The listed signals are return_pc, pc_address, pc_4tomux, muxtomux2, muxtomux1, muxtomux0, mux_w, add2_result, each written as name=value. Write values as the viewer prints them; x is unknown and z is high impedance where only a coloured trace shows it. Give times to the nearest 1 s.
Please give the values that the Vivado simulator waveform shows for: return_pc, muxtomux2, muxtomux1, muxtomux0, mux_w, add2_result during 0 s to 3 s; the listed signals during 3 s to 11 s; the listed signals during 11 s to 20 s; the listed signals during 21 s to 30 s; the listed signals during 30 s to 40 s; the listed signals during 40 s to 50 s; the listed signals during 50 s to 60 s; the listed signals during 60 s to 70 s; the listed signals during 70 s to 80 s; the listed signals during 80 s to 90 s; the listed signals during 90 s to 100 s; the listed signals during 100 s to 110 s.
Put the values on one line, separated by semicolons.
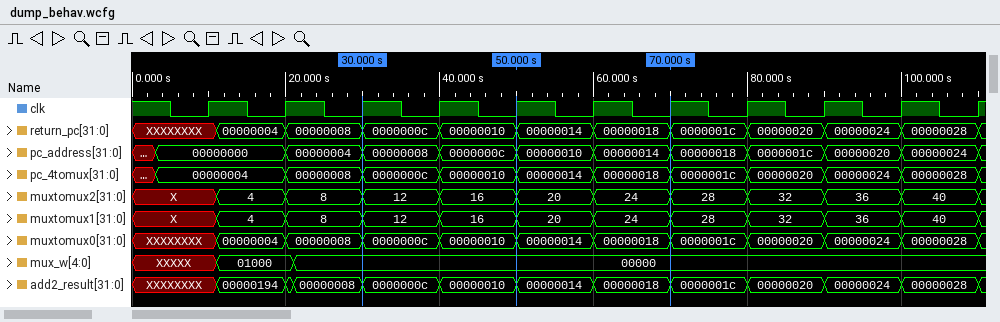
return_pc=XXXXXXXX, muxtomux2=X, muxtomux1=X, muxtomux0=XXXXXXXX, mux_w=XXXXX, add2_result=XXXXXXXX; return_pc=XXXXXXXX, pc_address=00000000, pc_4tomux=00000004, muxtomux2=X, muxtomux1=X, muxtomux0=XXXXXXXX, mux_w=XXXXX, add2_result=XXXXXXXX; return_pc=00000004, pc_address=00000000, pc_4tomux=00000004, muxtomux2=4, muxtomux1=4, muxtomux0=00000004, mux_w=01000, add2_result=00000194; return_pc=00000008, pc_address=00000004, pc_4tomux=00000008, muxtomux2=8, muxtomux1=8, muxtomux0=00000008, mux_w=00000, add2_result=00000008; return_pc=0000000c, pc_address=00000008, pc_4tomux=0000000c, muxtomux2=12, muxtomux1=12, muxtomux0=0000000c, mux_w=00000, add2_result=0000000c; return_pc=00000010, pc_address=0000000c, pc_4tomux=00000010, muxtomux2=16, muxtomux1=16, muxtomux0=00000010, mux_w=00000, add2_result=00000010; return_pc=00000014, pc_address=00000010, pc_4tomux=00000014, muxtomux2=20, muxtomux1=20, muxtomux0=00000014, mux_w=00000, add2_result=00000014; return_pc=00000018, pc_address=00000014, pc_4tomux=00000018, muxtomux2=24, muxtomux1=24, muxtomux0=00000018, mux_w=00000, add2_result=00000018; return_pc=0000001c, pc_address=00000018, pc_4tomux=0000001c, muxtomux2=28, muxtomux1=28, muxtomux0=0000001c, mux_w=00000, add2_result=0000001c; return_pc=00000020, pc_address=0000001c, pc_4tomux=00000020, muxtomux2=32, muxtomux1=32, muxtomux0=00000020, mux_w=00000, add2_result=00000020; return_pc=00000024, pc_address=00000020, pc_4tomux=00000024, muxtomux2=36, muxtomux1=36, muxtomux0=00000024, mux_w=00000, add2_result=00000024; return_pc=00000028, pc_address=00000024, pc_4tomux=00000028, muxtomux2=40, muxtomux1=40, muxtomux0=00000028, mux_w=00000, add2_result=00000028
